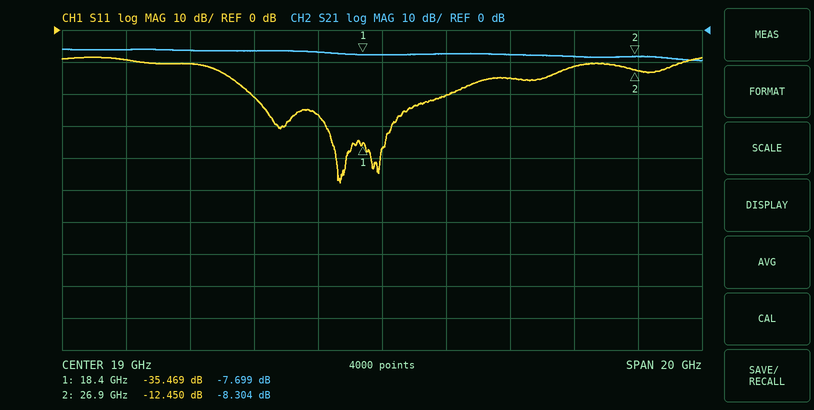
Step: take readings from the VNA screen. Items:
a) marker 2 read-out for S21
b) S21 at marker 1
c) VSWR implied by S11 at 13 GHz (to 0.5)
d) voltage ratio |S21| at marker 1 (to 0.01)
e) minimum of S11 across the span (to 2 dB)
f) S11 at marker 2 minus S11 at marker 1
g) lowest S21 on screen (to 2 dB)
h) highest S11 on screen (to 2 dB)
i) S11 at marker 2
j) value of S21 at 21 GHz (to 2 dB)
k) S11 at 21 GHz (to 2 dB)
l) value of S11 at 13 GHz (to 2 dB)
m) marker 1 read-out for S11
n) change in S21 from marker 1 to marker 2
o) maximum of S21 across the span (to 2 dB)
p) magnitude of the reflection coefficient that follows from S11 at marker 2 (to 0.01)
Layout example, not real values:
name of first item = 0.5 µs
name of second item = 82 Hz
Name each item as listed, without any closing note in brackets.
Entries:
marker 2 read-out for S21 = -8.304 dB
S21 at marker 1 = -7.699 dB
VSWR implied by S11 at 13 GHz = 2.0
voltage ratio |S21| at marker 1 = 0.41
minimum of S11 across the span = -48 dB
S11 at marker 2 minus S11 at marker 1 = 23.019 dB
lowest S21 on screen = -10 dB
highest S11 on screen = -8 dB
S11 at marker 2 = -12.450 dB
value of S21 at 21 GHz = -8 dB
S11 at 21 GHz = -20 dB
value of S11 at 13 GHz = -10 dB
marker 1 read-out for S11 = -35.469 dB
change in S21 from marker 1 to marker 2 = -0.605 dB
maximum of S21 across the span = -6 dB
magnitude of the reflection coefficient that follows from S11 at marker 2 = 0.24
